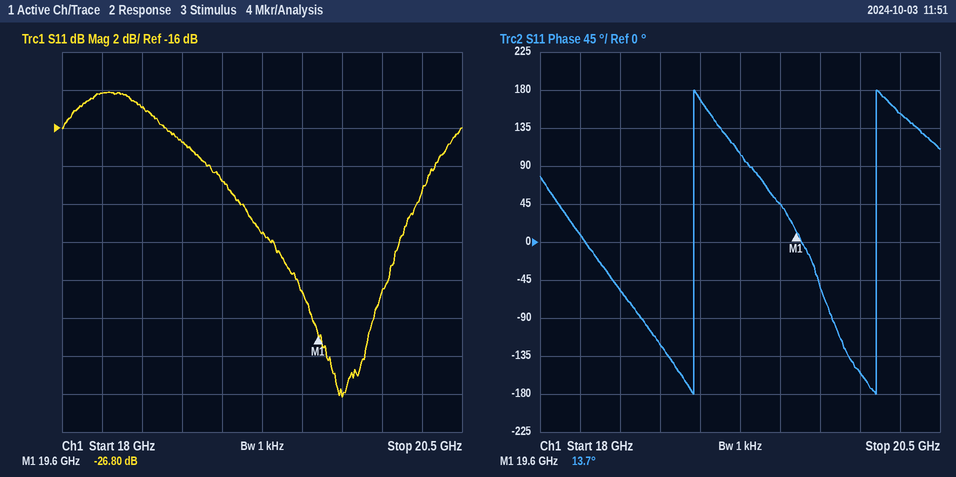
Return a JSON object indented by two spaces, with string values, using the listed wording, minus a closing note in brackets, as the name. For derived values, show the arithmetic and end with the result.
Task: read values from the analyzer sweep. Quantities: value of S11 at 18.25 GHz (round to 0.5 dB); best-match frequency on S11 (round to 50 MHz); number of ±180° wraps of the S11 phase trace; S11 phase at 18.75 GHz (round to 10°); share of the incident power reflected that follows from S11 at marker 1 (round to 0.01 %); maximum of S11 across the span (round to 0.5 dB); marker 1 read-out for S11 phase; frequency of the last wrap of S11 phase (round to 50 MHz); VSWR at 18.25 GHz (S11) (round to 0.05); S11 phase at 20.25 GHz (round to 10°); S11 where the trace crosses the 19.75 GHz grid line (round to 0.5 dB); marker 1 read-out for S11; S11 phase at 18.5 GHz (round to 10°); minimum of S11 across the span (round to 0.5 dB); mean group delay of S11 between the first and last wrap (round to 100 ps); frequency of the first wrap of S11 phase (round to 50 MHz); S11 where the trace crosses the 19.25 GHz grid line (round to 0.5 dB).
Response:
{
  "value of S11 at 18.25 GHz": "-14.0 dB",
  "best-match frequency on S11": "19.75 GHz",
  "number of ±180° wraps of the S11 phase trace": "2",
  "S11 phase at 18.75 GHz": "-120°",
  "share of the incident power reflected that follows from S11 at marker 1": "10^(-26.8/10) ≈ 0.21 %",
  "maximum of S11 across the span": "-14.0 dB",
  "marker 1 read-out for S11 phase": "13.7°",
  "frequency of the last wrap of S11 phase": "20.10 GHz",
  "VSWR at 18.25 GHz (S11)": "|Γ| = 10^(-14/20) = 0.1995; VSWR = (1 + 0.1995)/(1 − 0.1995) ≈ 1.50",
  "S11 phase at 20.25 GHz": "150°",
  "S11 where the trace crosses the 19.75 GHz grid line": "-30.0 dB",
  "marker 1 read-out for S11": "-26.80 dB",
  "S11 phase at 18.5 GHz": "-60°",
  "minimum of S11 across the span": "-30.0 dB",
  "mean group delay of S11 between the first and last wrap": "1 cycle / (20.10 GHz − 18.95 GHz) ≈ 870 ps, so 900 ps to the nearest 100 ps",
  "frequency of the first wrap of S11 phase": "18.95 GHz",
  "S11 where the trace crosses the 19.25 GHz grid line": "-21.5 dB"
}
